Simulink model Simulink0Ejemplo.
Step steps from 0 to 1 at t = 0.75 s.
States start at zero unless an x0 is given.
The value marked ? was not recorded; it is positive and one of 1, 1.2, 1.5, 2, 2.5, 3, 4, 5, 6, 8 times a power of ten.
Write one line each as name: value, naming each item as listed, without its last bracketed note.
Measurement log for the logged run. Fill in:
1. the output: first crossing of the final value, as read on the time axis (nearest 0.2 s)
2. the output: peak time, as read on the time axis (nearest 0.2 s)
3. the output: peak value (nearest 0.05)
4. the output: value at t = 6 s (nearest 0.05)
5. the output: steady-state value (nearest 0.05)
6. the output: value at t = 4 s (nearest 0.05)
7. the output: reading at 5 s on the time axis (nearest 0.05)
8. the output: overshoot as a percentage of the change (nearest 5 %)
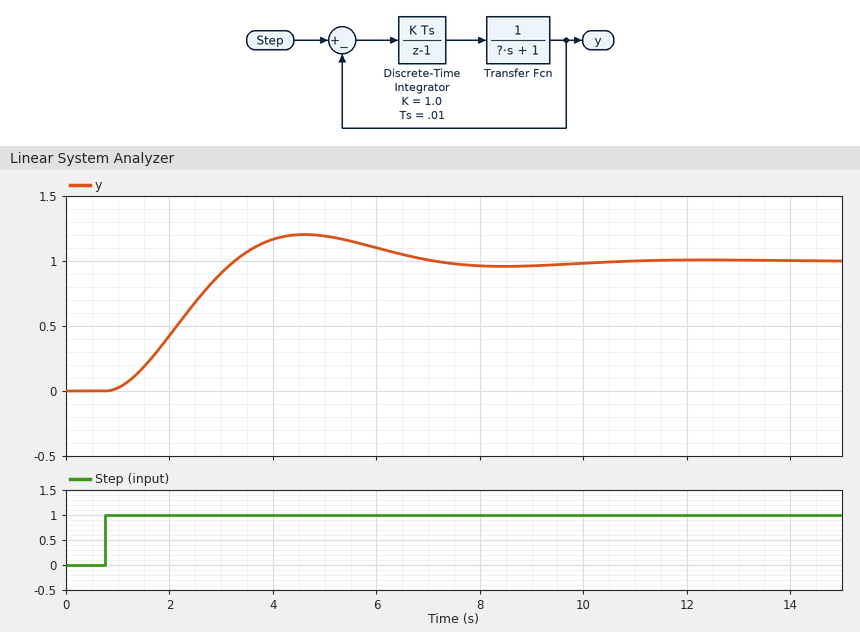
the output: first crossing of the final value, as read on the time axis: 3.2 s
the output: peak time, as read on the time axis: 4.6 s
the output: peak value: 1.20
the output: value at t = 6 s: 1.10
the output: steady-state value: 1.00
the output: value at t = 4 s: 1.15
the output: reading at 5 s on the time axis: 1.20
the output: overshoot as a percentage of the change: 20 %
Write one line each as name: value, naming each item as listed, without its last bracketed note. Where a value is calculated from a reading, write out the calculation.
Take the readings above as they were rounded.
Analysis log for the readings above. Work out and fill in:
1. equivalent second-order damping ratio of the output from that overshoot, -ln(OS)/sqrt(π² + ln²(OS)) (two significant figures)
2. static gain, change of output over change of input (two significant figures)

equivalent second-order damping ratio of the output from that overshoot, -ln(OS)/sqrt(π² + ln²(OS)): ln(0.2) = -1.609; 1.609 / sqrt(9.870 + 2.590) = 0.46
static gain, change of output over change of input: (1 - 0) / (1 - 0) = 1.0
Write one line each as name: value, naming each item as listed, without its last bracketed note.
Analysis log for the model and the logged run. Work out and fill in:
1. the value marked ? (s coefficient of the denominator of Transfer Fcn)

the value marked ?: 1.2
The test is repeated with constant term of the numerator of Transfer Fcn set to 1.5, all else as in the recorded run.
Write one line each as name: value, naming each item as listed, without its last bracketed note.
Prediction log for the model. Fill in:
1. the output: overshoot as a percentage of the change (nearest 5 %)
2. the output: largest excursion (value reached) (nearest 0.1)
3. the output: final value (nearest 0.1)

the output: overshoot as a percentage of the change: 30 %
the output: largest excursion (value reached): 1.3
the output: final value: 1.0
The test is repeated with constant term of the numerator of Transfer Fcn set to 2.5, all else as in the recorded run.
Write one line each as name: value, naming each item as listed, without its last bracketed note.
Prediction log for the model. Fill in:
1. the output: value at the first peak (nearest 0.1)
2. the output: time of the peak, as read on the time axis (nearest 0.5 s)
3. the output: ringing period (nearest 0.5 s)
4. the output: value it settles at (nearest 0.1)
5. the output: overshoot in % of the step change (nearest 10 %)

the output: value at the first peak: 1.4
the output: time of the peak, as read on the time axis: 3.0 s
the output: ringing period: 4.5 s
the output: value it settles at: 1.0
the output: overshoot in % of the step change: 40 %
